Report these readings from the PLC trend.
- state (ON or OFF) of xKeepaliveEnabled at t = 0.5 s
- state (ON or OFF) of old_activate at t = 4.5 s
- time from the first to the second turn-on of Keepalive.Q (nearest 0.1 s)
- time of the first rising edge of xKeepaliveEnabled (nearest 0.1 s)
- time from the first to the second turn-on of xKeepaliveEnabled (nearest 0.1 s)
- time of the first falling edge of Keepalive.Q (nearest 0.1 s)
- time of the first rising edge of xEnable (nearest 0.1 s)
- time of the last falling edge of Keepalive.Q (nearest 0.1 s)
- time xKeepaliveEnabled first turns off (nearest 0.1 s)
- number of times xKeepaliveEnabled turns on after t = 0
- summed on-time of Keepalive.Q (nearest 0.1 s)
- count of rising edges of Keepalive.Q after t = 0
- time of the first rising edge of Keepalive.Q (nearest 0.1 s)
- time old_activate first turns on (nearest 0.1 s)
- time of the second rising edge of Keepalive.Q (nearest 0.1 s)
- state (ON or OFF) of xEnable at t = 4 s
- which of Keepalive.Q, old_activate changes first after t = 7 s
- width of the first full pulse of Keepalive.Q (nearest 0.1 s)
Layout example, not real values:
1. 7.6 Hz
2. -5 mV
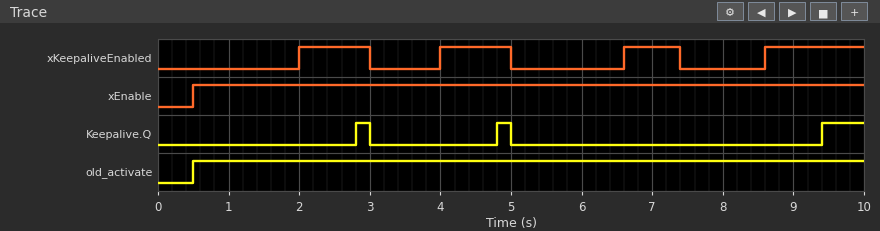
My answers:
1. OFF
2. ON
3. 2.0 s
4. 2.0 s
5. 2.0 s
6. 3.0 s
7. 0.5 s
8. 5.0 s
9. 3.0 s
10. 4
11. 1.0 s
12. 3
13. 2.8 s
14. 0.5 s
15. 4.8 s
16. ON
17. Keepalive.Q
18. 0.2 s
